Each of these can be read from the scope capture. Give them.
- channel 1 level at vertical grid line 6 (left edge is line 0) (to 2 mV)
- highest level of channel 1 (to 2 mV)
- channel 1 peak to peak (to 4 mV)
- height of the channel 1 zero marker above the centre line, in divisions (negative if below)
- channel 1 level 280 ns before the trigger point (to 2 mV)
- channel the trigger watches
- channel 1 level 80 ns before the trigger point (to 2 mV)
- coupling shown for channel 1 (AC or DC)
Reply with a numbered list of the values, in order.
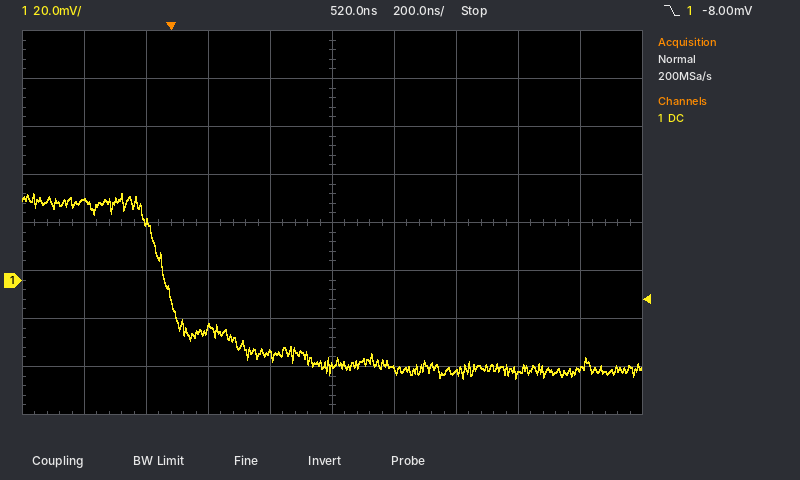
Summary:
1. -38 mV
2. 36 mV
3. 76 mV
4. -1.2 div
5. 34 mV
6. channel 1
7. 24 mV
8. DC
